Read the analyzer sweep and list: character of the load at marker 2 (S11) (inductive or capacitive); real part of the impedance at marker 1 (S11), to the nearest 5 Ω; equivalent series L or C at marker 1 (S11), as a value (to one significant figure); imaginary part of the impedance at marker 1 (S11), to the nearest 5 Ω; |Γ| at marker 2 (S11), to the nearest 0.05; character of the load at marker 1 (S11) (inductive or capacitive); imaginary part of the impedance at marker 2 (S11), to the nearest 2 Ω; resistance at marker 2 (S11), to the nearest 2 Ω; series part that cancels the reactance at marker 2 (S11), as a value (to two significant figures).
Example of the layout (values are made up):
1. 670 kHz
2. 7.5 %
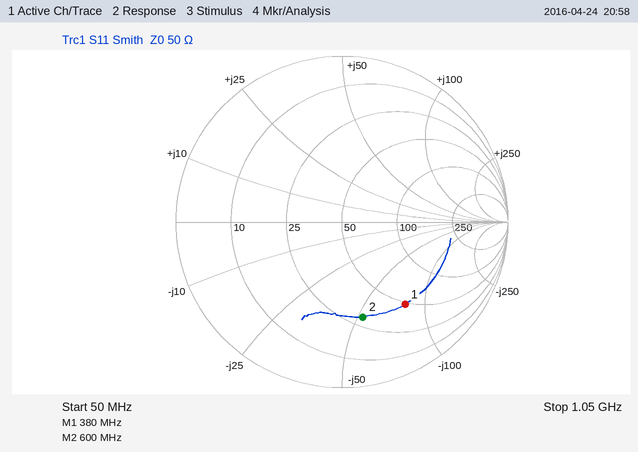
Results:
1. capacitive
2. 50 Ω
3. 5 pF
4. -80 Ω
5. 0.60
6. capacitive
7. -52 Ω
8. 30 Ω
9. 14 nH
